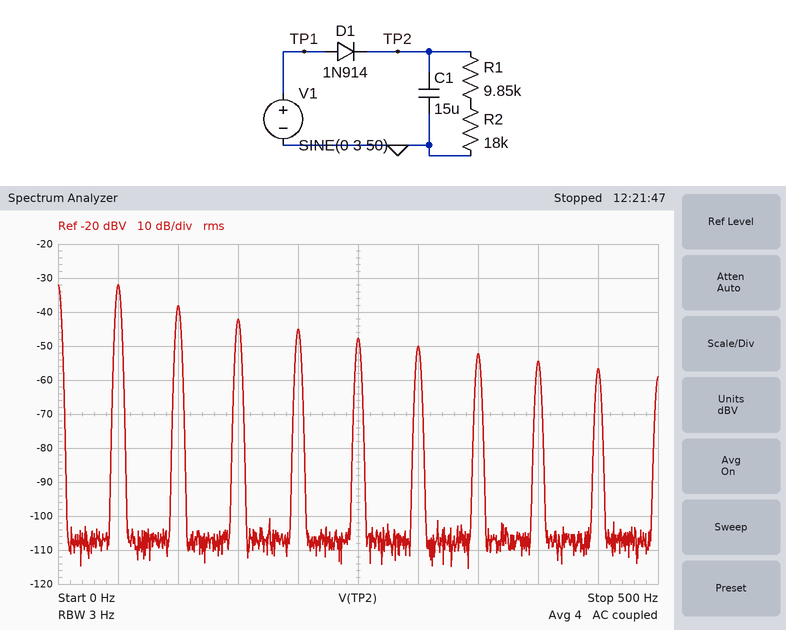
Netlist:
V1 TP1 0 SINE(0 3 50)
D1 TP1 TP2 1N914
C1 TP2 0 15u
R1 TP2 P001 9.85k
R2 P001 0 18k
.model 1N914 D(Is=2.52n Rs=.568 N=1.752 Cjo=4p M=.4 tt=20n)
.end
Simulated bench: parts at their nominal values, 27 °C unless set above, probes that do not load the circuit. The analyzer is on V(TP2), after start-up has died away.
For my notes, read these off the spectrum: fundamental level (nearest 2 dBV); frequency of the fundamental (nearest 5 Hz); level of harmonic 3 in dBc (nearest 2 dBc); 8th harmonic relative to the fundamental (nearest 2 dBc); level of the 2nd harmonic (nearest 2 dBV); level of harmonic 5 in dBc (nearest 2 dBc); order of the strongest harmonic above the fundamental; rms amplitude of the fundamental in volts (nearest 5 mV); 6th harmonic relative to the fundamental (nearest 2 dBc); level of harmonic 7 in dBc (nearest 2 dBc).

-32 dBV
50 Hz
-10 dBc
-22 dBc
-38 dBV
-16 dBc
2
25 mV
-18 dBc
-20 dBc
